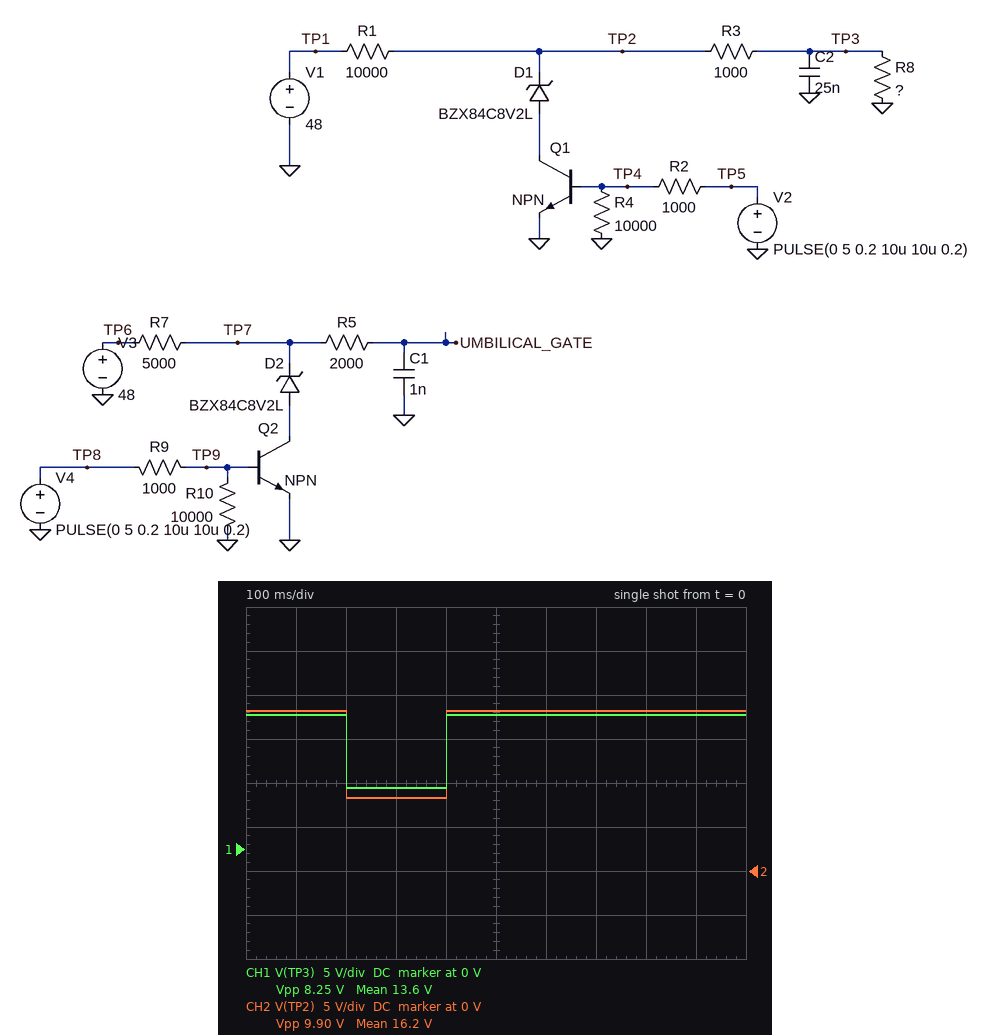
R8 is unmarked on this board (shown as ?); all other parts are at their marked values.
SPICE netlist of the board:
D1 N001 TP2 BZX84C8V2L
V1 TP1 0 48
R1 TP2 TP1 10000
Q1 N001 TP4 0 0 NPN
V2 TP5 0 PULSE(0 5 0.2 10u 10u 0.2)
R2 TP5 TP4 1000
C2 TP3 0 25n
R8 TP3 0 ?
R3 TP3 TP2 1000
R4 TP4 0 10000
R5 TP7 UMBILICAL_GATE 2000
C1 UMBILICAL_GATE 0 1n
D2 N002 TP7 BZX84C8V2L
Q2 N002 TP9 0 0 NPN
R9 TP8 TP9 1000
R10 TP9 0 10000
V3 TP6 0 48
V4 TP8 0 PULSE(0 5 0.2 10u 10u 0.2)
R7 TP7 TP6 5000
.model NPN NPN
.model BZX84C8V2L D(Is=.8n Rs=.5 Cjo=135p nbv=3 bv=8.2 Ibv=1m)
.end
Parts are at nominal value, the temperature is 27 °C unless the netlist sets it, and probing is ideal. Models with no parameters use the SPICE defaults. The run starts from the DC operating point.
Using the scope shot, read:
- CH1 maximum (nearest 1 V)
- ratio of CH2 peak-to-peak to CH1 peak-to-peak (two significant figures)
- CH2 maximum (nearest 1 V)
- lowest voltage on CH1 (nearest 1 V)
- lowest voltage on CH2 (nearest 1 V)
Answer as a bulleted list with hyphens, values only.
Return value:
- 15 V
- 1.2
- 18 V
- 7 V
- 8 V
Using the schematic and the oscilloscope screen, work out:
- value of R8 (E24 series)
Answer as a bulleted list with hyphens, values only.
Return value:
- 5.1 kΩ
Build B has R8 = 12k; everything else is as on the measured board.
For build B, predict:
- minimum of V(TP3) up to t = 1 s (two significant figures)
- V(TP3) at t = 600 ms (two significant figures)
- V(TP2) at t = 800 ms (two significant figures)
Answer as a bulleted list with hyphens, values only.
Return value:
- 7.7 V
- 25 V
- 27 V
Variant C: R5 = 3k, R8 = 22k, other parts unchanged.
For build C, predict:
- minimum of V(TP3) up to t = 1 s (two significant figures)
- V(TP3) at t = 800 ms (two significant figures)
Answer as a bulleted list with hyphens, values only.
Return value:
- 8.0 V
- 32 V
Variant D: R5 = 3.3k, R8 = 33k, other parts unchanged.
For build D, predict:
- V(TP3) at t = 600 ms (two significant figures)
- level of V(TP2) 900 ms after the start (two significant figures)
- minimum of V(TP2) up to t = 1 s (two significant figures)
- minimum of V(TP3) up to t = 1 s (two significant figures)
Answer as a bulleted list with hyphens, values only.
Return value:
- 36 V
- 37 V
- 8.3 V
- 8.1 V
